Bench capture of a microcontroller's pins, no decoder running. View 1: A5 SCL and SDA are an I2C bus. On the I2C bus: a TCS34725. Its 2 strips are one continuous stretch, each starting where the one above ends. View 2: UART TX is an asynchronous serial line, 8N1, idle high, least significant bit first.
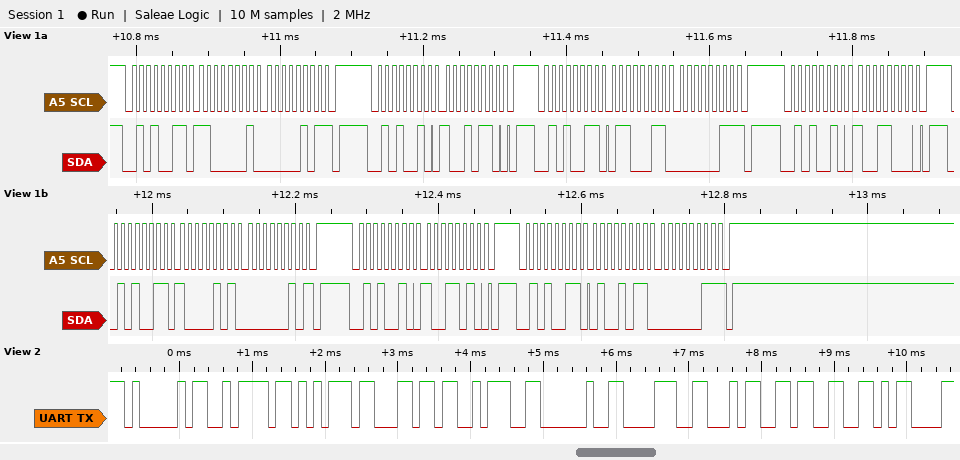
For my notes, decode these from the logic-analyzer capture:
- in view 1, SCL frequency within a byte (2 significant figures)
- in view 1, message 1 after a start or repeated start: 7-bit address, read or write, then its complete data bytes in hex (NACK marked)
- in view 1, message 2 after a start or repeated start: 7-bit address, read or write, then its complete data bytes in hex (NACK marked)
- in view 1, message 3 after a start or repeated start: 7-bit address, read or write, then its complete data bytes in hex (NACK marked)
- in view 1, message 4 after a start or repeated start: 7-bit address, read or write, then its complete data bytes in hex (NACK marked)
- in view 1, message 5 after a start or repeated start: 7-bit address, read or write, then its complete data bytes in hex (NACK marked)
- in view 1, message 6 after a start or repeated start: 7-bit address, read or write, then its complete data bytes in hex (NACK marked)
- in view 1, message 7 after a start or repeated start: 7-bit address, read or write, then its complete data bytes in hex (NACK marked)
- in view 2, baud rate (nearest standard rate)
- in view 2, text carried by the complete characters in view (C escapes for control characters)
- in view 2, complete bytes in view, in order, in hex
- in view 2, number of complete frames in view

100 kHz
0x29 read: C1 05 NACK
0x29 write: 96
0x29 read: 63 03 NACK
0x29 write: 98
0x29 read: 85 02 NACK
0x29 write: 9A
0x29 read: 4B 03 NACK
9600 baud
"Azul: 843\r"
41 7A 75 6C 3A 20 38 34 33 0D
10
